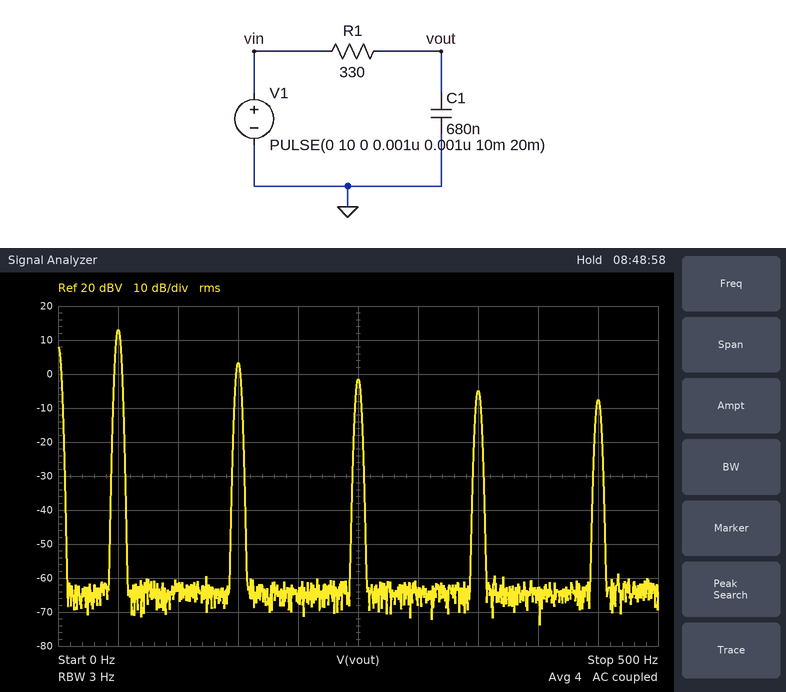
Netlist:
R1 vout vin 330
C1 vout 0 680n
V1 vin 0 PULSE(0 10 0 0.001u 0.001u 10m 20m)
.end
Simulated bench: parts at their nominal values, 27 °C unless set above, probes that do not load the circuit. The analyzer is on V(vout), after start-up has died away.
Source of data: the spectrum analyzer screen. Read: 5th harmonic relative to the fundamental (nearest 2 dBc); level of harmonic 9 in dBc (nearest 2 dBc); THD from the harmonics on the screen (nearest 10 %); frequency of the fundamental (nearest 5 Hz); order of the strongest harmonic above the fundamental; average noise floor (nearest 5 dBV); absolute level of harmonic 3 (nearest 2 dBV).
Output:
-14 dBc
-20 dBc
40 %
50 Hz
3
-65 dBV
4 dBV
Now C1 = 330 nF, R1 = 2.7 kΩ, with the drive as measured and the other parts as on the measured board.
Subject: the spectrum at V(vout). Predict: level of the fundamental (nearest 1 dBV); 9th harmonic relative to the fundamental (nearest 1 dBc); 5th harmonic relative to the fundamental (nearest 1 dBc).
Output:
13 dBV
-27 dBc
-18 dBc
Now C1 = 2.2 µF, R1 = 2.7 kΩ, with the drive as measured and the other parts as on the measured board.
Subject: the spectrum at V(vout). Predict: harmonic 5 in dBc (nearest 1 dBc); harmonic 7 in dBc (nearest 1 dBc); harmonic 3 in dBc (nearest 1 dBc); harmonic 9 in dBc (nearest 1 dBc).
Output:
-27 dBc
-33 dBc
-18 dBc
-37 dBc
